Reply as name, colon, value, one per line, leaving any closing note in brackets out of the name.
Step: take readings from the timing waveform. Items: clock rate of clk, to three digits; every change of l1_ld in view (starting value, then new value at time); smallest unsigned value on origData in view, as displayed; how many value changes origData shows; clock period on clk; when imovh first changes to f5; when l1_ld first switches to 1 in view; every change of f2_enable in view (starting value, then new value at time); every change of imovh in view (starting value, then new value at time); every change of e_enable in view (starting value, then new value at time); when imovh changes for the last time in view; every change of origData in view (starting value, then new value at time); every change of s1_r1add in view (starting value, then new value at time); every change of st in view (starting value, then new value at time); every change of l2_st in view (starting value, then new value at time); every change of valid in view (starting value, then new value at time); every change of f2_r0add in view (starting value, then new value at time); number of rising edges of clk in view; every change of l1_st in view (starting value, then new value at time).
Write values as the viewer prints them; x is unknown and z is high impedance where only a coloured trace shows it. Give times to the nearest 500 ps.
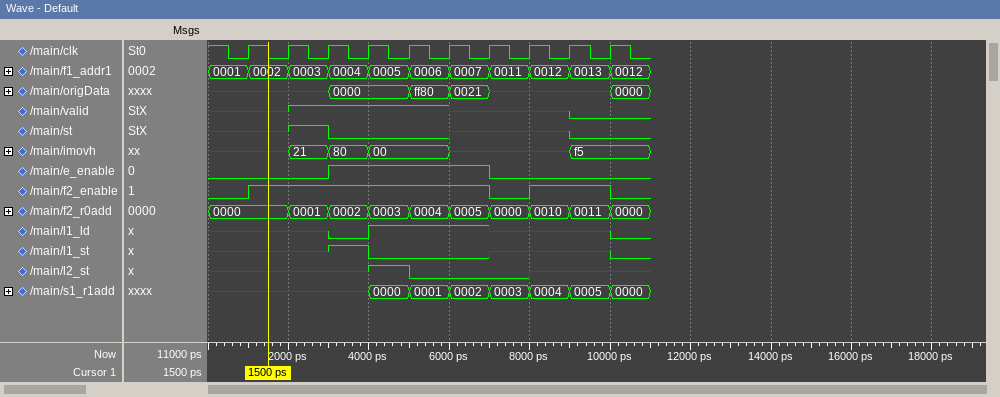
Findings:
clock rate of clk, to three digits: 1.00 GHz
every change of l1_ld in view: x, 0 at 3000 ps, 1 at 4000 ps, x at 7000 ps, 0 at 10000 ps
smallest unsigned value on origData in view, as displayed: 0000
how many value changes origData shows: 5
clock period on clk: 1000 ps
when imovh first changes to f5: 9000 ps
when l1_ld first switches to 1 in view: 4000 ps
every change of f2_enable in view: 0, 1 at 1000 ps, 0 at 7000 ps, 1 at 8000 ps, 0 at 10000 ps
every change of imovh in view: x, 21 at 2000 ps, 80 at 3000 ps, 00 at 4000 ps, x at 6000 ps, f5 at 9000 ps
every change of e_enable in view: 0, 1 at 3000 ps, 0 at 7000 ps
when imovh changes for the last time in view: 9000 ps
every change of origData in view: x, 0000 at 3000 ps, ff80 at 5000 ps, 0021 at 6000 ps, x at 7000 ps, 0000 at 10000 ps
every change of s1_r1add in view: x, 0000 at 4000 ps, 0001 at 5000 ps, 0002 at 6000 ps, 0003 at 7000 ps, 0004 at 8000 ps, 0005 at 9000 ps, 0000 at 10000 ps
every change of st in view: x, 1 at 2000 ps, 0 at 3000 ps, x at 6000 ps, 0 at 9000 ps
every change of l2_st in view: x, 1 at 4000 ps, 0 at 5000 ps, x at 8000 ps
every change of valid in view: x, 1 at 2000 ps, x at 6000 ps, 0 at 9000 ps
every change of f2_r0add in view: 0000, 0001 at 2000 ps, 0002 at 3000 ps, 0003 at 4000 ps, 0004 at 5000 ps, 0005 at 6000 ps, 0000 at 7000 ps, 0010 at 8000 ps, 0011 at 9000 ps, 0000 at 10000 ps
number of rising edges of clk in view: 10
every change of l1_st in view: x, 1 at 3000 ps, 0 at 4000 ps, x at 7000 ps, 0 at 10000 ps
